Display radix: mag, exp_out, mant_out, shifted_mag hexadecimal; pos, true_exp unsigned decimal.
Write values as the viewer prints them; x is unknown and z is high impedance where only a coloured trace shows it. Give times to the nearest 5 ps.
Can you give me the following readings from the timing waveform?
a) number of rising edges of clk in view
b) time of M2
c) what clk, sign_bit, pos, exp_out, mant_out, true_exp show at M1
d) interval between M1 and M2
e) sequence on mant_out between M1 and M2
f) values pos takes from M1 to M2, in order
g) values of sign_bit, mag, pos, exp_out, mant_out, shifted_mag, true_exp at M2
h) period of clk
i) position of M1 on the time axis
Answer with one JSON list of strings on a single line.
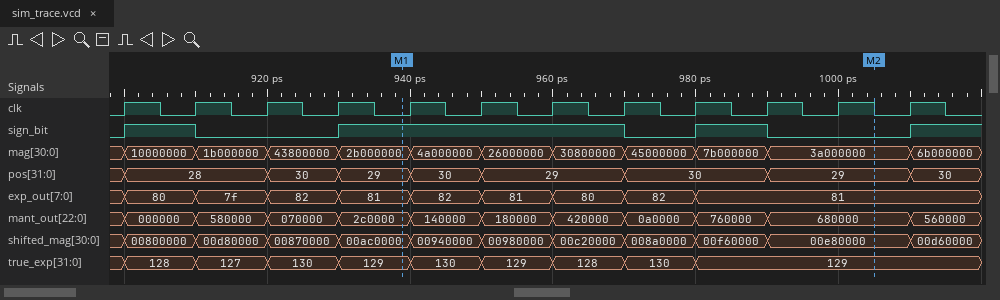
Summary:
["12", "1005 ps", "clk=0, sign_bit=1, pos=29, exp_out=81, mant_out=2c0000, true_exp=129", "65 ps", "2c0000, 140000, 180000, 420000, 0a0000, 760000, 680000", "29, 30, 29, 30, 29", "sign_bit=0, mag=3a000000, pos=29, exp_out=81, mant_out=680000, shifted_mag=00e80000, true_exp=129", "10 ps", "940 ps"]
